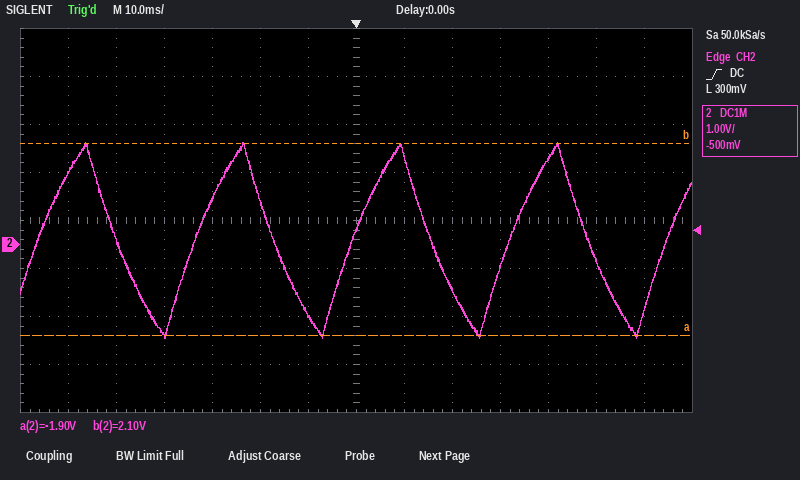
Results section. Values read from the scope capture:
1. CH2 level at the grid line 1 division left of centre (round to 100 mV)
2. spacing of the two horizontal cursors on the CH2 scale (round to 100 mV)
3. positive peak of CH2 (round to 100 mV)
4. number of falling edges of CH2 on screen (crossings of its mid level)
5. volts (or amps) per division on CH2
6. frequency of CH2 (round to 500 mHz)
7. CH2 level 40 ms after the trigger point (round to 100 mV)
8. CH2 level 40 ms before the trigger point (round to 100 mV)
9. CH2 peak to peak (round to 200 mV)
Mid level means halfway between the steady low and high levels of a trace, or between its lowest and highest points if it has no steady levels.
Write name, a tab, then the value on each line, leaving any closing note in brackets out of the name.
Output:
CH2 level at the grid line 1 division left of centre	-1.5 V
spacing of the two horizontal cursors on the CH2 scale	4.0 V
positive peak of CH2	2.1 V
number of falling edges of CH2 on screen	4
volts (or amps) per division on CH2	1 V
frequency of CH2	30.5 Hz
CH2 level 40 ms after the trigger point	1.8 V
CH2 level 40 ms before the trigger point	-1.9 V
CH2 peak to peak	4.0 V
